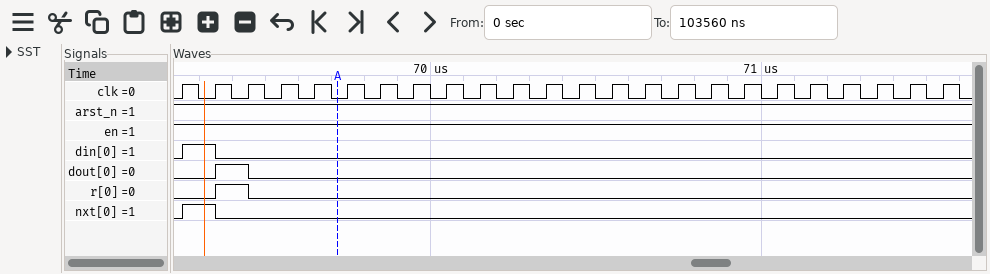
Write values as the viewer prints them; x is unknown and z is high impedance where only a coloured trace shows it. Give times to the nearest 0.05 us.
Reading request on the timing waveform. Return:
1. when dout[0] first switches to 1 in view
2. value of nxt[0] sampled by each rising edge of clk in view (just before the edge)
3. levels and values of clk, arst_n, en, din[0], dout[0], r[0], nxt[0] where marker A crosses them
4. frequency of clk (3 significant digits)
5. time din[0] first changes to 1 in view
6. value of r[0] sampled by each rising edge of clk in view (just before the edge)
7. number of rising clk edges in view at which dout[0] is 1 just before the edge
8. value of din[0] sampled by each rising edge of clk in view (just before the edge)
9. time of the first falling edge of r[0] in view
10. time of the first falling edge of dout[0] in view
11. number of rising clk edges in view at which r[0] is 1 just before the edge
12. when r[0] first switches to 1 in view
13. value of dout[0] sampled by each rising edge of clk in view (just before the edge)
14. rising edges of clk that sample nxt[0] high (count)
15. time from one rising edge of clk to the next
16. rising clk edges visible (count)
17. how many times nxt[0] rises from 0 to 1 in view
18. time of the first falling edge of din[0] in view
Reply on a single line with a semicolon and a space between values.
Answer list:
69.35 us; 0 1 0 0 0 0 0 0 0 0 0 0 0 0 0 0 0 0 0 0 0 0 0 0; clk=0, arst_n=1, en=1, din[0]=0, dout[0]=0, r[0]=0, nxt[0]=0; 10.0 MHz; 69.25 us; 0 0 1 0 0 0 0 0 0 0 0 0 0 0 0 0 0 0 0 0 0 0 0 0; 1; 0 1 0 0 0 0 0 0 0 0 0 0 0 0 0 0 0 0 0 0 0 0 0 0; 69.45 us; 69.45 us; 1; 69.35 us; 0 0 1 0 0 0 0 0 0 0 0 0 0 0 0 0 0 0 0 0 0 0 0 0; 1; 0.1 us; 24; 1; 69.35 us
